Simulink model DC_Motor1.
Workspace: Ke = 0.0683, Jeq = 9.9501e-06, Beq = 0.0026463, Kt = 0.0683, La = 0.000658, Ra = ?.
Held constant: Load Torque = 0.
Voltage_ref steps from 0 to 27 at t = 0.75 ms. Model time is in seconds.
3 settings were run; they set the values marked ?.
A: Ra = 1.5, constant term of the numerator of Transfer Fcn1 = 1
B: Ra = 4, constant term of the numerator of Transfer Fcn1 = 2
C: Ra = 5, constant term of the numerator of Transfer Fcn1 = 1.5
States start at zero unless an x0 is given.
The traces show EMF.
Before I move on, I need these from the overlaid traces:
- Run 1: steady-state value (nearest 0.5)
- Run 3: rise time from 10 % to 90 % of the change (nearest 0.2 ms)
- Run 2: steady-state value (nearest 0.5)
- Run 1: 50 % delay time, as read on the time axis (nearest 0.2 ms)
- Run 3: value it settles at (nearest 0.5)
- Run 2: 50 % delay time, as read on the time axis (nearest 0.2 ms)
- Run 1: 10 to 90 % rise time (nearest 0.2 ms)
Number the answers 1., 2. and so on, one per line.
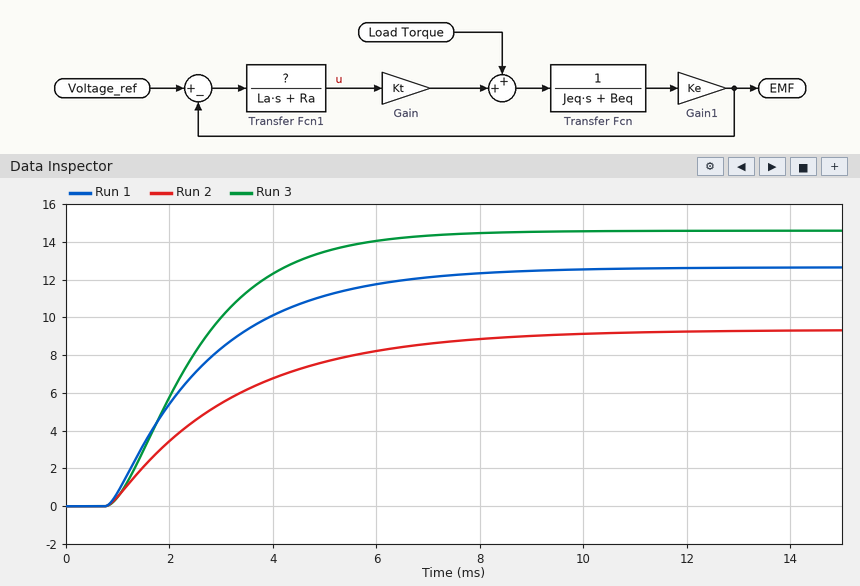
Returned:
1. 12.5
2. 3.4 ms
3. 9.5
4. 2.2 ms
5. 14.5
6. 2.6 ms
7. 4.2 ms
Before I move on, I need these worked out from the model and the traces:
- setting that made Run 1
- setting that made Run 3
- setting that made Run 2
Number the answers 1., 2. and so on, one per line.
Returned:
1. B
2. A
3. C
